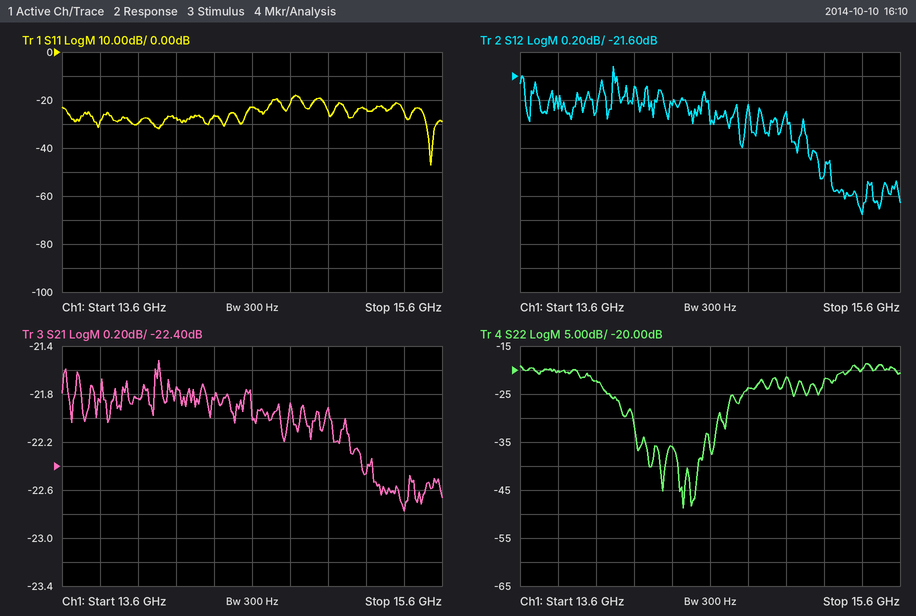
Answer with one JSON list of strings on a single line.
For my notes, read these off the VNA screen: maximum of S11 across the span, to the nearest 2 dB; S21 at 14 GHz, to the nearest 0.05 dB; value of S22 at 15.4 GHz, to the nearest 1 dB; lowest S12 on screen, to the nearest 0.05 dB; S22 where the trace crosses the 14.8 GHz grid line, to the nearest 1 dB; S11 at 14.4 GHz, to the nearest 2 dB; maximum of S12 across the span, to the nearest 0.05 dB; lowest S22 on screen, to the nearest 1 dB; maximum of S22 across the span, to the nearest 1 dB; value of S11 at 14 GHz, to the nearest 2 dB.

["-18 dB", "-21.85 dB", "-20 dB", "-22.75 dB", "-24 dB", "-26 dB", "-21.50 dB", "-49 dB", "-19 dB", "-30 dB"]
